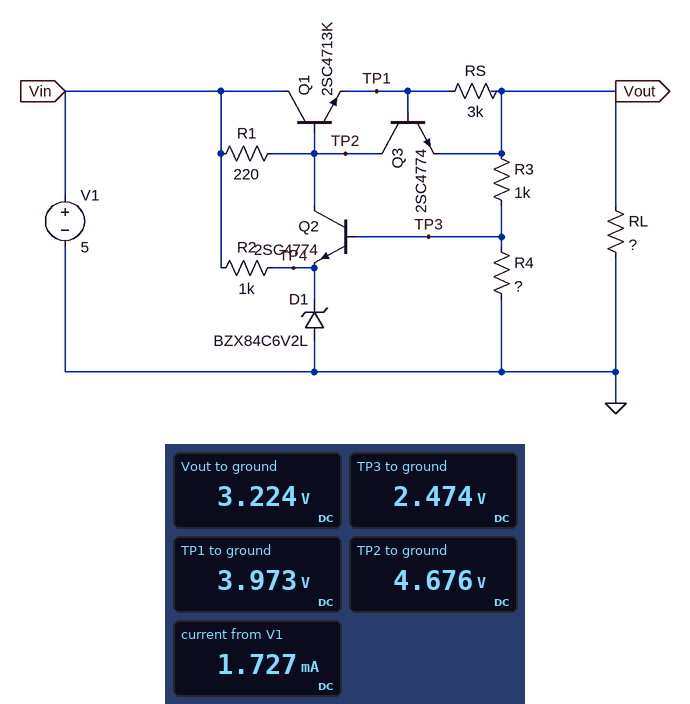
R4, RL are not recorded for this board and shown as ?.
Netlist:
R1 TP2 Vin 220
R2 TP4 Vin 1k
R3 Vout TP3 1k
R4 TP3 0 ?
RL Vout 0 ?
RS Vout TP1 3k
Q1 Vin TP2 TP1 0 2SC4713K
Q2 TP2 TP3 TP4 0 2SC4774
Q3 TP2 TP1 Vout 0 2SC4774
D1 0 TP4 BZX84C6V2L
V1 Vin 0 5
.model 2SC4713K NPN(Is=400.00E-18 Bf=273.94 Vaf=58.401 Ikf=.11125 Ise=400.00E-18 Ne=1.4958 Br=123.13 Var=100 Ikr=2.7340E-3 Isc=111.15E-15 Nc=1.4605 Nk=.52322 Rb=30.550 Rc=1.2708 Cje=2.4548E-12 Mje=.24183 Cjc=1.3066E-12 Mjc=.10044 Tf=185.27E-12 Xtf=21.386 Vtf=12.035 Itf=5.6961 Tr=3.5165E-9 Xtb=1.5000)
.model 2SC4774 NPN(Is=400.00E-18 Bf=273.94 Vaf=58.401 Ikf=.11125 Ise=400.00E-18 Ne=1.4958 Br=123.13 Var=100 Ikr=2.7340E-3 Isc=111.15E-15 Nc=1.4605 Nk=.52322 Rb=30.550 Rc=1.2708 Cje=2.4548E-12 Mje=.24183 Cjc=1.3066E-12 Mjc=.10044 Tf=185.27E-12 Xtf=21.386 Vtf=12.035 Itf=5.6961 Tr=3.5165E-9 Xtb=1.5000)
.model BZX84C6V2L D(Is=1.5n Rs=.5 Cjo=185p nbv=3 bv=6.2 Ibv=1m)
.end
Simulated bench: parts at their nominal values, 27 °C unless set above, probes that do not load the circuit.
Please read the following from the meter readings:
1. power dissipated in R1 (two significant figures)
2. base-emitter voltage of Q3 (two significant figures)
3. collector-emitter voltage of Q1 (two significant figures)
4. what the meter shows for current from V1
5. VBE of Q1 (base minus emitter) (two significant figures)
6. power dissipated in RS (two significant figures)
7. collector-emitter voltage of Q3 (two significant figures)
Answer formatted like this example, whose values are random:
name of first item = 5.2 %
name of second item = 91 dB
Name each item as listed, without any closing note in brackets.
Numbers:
power dissipated in R1 = 480 µW
base-emitter voltage of Q3 = 750 mV
collector-emitter voltage of Q1 = 1.0 V
what the meter shows for current from V1 = 1.727 mA
VBE of Q1 (base minus emitter) = 700 mV
power dissipated in RS = 190 µW
collector-emitter voltage of Q3 = 1.5 V
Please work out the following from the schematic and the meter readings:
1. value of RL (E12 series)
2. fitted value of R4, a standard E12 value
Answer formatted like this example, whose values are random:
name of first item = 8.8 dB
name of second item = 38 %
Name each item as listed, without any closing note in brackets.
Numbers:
value of RL = 3.3 kΩ
fitted value of R4, a standard E12 value = 3.3 kΩ
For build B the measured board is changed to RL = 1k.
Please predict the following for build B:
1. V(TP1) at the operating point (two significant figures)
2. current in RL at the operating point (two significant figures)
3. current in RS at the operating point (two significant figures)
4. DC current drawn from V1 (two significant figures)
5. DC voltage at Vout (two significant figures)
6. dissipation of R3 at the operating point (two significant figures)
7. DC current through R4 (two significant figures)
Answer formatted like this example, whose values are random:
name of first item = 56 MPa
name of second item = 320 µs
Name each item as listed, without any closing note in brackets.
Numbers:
V(TP1) at the operating point = 3.6 V
current in RL at the operating point = 2.8 mA
current in RS at the operating point = 260 µA
DC current drawn from V1 = 3.5 mA
DC voltage at Vout = 2.8 V
dissipation of R3 at the operating point = 430 µW
DC current through R4 = 660 µA
